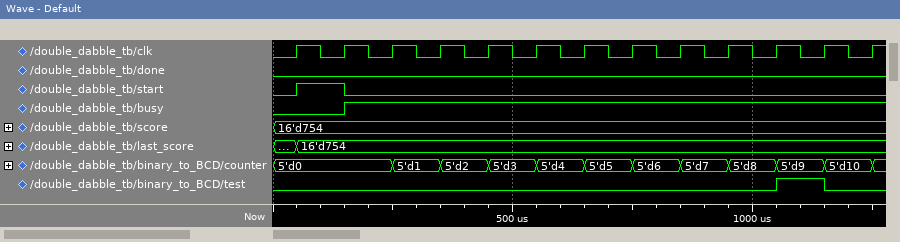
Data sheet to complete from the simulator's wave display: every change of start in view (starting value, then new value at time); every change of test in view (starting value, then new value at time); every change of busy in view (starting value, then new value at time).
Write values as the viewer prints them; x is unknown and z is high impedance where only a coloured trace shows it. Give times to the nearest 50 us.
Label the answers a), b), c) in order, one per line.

a) 0, 1 at 50 us, 0 at 150 us
b) 0, 1 at 1050 us, 0 at 1150 us
c) 0, 1 at 150 us
